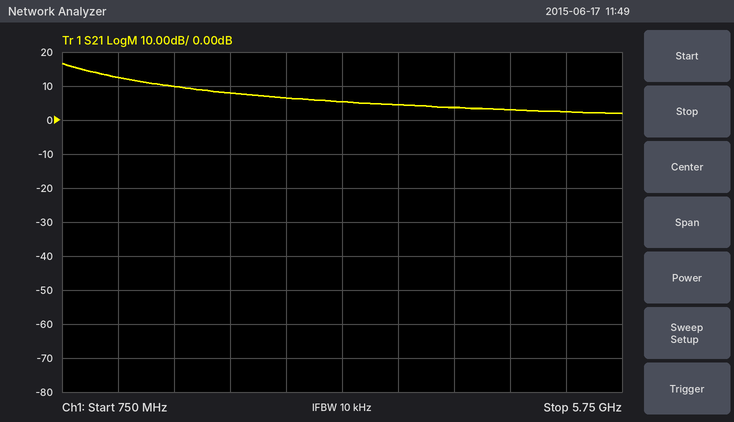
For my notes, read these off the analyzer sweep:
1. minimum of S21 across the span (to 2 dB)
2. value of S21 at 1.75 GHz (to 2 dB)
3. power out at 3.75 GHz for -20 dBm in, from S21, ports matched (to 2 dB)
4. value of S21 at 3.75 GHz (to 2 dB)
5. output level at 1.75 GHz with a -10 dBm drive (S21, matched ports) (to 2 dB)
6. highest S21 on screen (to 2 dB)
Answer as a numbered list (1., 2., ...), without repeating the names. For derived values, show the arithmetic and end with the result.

1. 2 dB
2. 10 dB
3. -20 dBm + (4 dB) = -16 dBm
4. 4 dB
5. -10 dBm + (10 dB) = 0 dBm
6. 16 dB
